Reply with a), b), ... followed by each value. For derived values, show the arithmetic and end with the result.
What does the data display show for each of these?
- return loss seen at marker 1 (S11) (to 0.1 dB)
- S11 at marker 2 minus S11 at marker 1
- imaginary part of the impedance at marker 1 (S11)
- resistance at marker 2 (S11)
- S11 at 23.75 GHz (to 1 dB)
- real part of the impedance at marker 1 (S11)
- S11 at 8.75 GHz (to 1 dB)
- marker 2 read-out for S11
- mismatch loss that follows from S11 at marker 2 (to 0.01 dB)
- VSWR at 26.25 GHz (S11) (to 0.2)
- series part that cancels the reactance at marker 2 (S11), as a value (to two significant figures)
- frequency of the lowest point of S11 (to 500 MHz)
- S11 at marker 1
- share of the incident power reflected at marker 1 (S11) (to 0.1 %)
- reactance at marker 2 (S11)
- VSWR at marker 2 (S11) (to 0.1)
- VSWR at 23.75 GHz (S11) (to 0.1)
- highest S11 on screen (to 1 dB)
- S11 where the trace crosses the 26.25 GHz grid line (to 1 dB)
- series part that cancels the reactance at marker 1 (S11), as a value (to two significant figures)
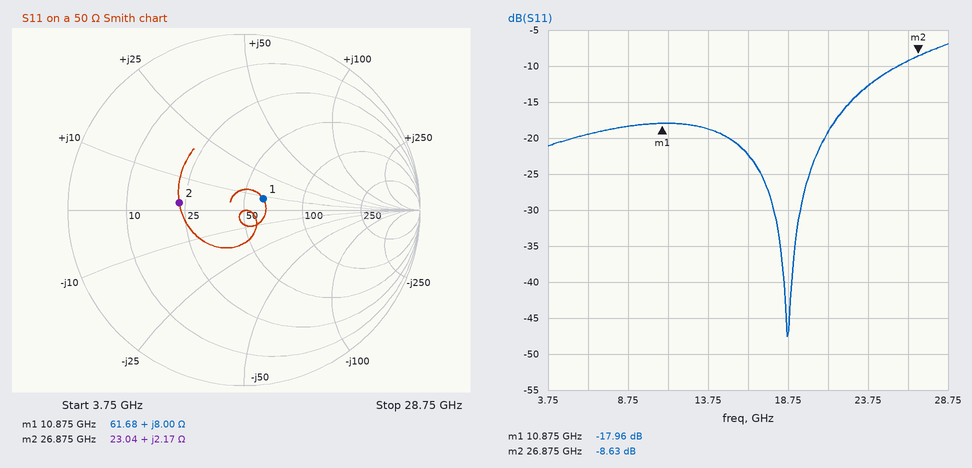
a) 18.0 dB
b) -8.63 − (-17.96) = 9.33 dB
c) +8.00 Ω
d) 23.04 Ω
e) -13 dB
f) 61.68 Ω
g) -18 dB
h) -8.63 dB
i) −10 log10(1 − 10^(-8.63/10)) ≈ 0.64 dB
j) |Γ| = 10^(-9/20) = 0.3548; VSWR = (1 + 0.3548)/(1 − 0.3548) ≈ 2.10, so 2.0 to the nearest 0.2
k) C = 1/(2π × 26.875 GHz × 2.17 Ω) ≈ 2.7 pF
l) 18.5 GHz
m) -17.96 dB
n) 10^(-17.96/10) ≈ 1.6 %
o) +2.17 Ω
p) 2.2
q) |Γ| = 10^(-13/20) = 0.2239; VSWR = (1 + 0.2239)/(1 − 0.2239) ≈ 1.6
r) -7 dB
s) -9 dB
t) C = 1/(2π × 10.875 GHz × 8 Ω) ≈ 1.8 pF
